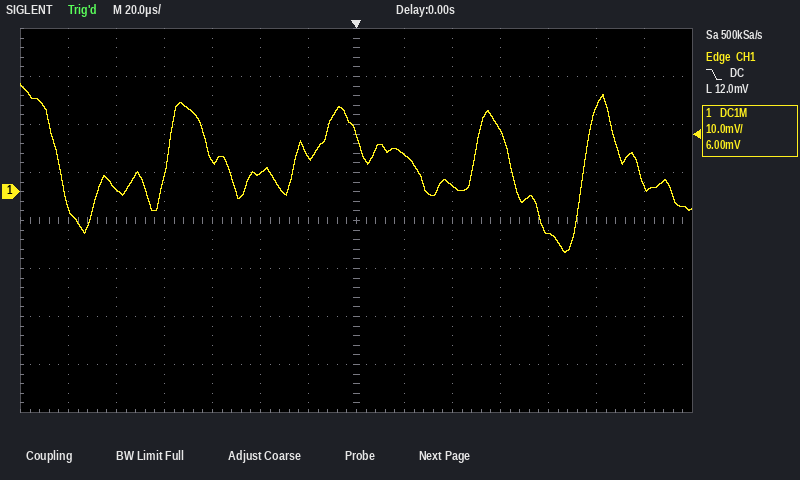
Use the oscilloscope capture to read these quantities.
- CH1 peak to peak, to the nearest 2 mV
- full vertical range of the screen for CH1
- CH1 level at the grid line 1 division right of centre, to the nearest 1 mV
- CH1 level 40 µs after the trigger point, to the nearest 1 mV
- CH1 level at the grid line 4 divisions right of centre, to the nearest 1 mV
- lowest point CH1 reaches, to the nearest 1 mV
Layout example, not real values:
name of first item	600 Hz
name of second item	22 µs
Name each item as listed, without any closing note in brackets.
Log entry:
CH1 peak to peak, to the nearest 2 mV	36 mV
full vertical range of the screen for CH1	80 mV
CH1 level at the grid line 1 division right of centre, to the nearest 1 mV	8 mV
CH1 level 40 µs after the trigger point, to the nearest 1 mV	1 mV
CH1 level at the grid line 4 divisions right of centre, to the nearest 1 mV	-9 mV
lowest point CH1 reaches, to the nearest 1 mV	-13 mV
